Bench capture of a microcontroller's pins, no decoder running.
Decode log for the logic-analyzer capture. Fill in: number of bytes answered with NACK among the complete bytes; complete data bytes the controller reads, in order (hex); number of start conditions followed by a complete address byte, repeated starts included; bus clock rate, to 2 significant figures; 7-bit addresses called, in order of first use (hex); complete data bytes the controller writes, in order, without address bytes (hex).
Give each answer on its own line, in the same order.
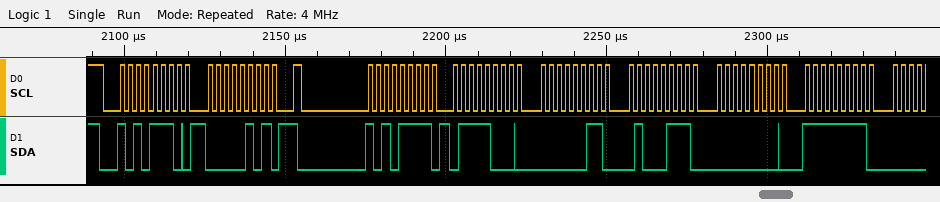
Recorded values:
0
78 03 47 00 FF
2
400 kHz
0x57
05
